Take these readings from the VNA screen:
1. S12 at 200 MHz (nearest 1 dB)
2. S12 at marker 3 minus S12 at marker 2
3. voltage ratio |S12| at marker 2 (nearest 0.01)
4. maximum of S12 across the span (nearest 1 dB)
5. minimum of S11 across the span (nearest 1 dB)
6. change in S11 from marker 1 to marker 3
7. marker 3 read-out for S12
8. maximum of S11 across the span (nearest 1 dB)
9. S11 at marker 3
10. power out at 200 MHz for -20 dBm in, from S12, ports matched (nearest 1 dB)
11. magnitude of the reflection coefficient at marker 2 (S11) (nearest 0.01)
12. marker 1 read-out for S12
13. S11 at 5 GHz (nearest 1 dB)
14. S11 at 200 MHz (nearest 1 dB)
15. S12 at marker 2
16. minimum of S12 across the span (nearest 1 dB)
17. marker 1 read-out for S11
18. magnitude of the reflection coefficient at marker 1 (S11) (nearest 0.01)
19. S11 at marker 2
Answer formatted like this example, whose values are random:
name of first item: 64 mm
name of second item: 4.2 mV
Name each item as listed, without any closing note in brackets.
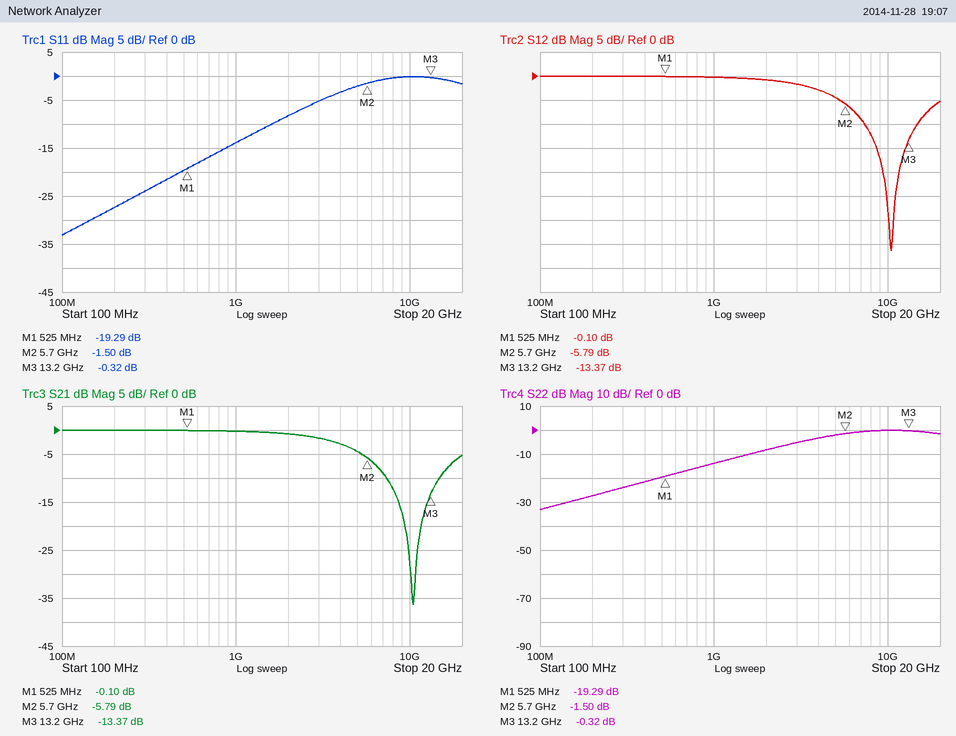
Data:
S12 at 200 MHz: 0 dB
S12 at marker 3 minus S12 at marker 2: -7.58 dB
voltage ratio |S12| at marker 2: 0.51
maximum of S12 across the span: 0 dB
minimum of S11 across the span: -33 dB
change in S11 from marker 1 to marker 3: 18.97 dB
marker 3 read-out for S12: -13.37 dB
maximum of S11 across the span: 0 dB
S11 at marker 3: -0.32 dB
power out at 200 MHz for -20 dBm in, from S12, ports matched: -20 dBm
magnitude of the reflection coefficient at marker 2 (S11): 0.84
marker 1 read-out for S12: -0.10 dB
S11 at 5 GHz: -2 dB
S11 at 200 MHz: -27 dB
S12 at marker 2: -5.79 dB
minimum of S12 across the span: -36 dB
marker 1 read-out for S11: -19.29 dB
magnitude of the reflection coefficient at marker 1 (S11): 0.11
S11 at marker 2: -1.50 dB
